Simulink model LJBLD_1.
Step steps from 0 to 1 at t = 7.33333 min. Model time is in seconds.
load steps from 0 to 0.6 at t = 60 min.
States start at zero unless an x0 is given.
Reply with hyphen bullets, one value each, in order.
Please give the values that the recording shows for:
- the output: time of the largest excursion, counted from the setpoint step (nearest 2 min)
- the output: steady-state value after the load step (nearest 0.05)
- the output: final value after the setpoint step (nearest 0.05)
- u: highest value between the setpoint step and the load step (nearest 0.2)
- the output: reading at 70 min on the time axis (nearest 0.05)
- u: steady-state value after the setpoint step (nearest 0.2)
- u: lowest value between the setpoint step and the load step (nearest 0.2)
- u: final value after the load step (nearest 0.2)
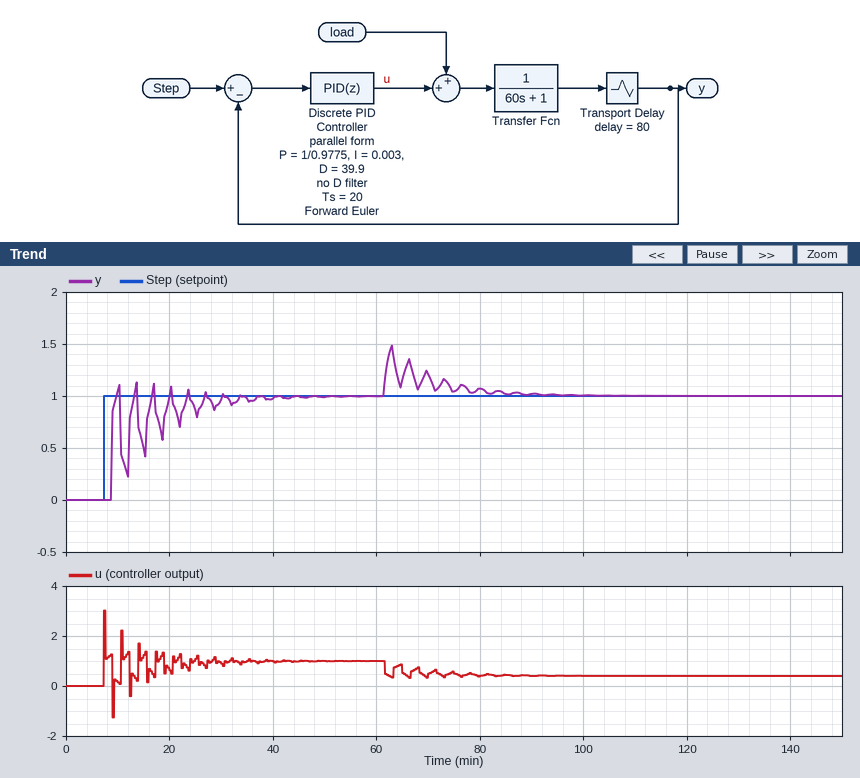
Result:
- 6 min
- 1.00
- 1.00
- 3.0
- 1.20
- 1.0
- -1.2
- 0.4
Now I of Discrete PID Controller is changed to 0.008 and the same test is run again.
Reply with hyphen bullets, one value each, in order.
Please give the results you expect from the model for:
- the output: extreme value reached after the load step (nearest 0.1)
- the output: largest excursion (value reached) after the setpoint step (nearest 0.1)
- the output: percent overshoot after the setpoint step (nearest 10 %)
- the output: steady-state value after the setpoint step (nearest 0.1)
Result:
- 1.5
- 1.3
- 30 %
- 1.0
